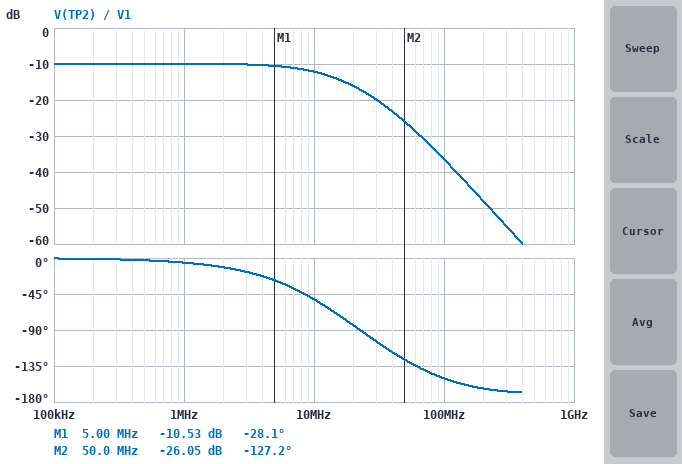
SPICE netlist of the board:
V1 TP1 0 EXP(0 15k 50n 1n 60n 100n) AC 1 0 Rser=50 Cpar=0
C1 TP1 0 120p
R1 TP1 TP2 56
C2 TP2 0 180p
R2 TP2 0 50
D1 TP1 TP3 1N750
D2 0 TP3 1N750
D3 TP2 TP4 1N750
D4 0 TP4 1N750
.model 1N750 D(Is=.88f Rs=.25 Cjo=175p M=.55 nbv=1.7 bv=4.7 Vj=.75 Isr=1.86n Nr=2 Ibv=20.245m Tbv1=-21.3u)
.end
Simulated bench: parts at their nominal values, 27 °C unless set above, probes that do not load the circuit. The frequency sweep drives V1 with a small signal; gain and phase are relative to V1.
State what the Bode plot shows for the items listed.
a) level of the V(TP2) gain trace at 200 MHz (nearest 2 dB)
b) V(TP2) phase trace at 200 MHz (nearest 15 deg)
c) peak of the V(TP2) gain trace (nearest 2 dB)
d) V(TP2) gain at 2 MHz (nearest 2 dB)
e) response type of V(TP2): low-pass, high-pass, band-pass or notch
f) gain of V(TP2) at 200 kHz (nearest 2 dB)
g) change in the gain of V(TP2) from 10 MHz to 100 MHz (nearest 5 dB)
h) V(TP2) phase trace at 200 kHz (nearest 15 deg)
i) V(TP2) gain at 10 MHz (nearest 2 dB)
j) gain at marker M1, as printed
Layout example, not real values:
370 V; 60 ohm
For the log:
-48 dB; -165 deg; -10 dB; -10 dB; low-pass; -10 dB; -25 dB; 0 deg; -12 dB; -10.53 dB
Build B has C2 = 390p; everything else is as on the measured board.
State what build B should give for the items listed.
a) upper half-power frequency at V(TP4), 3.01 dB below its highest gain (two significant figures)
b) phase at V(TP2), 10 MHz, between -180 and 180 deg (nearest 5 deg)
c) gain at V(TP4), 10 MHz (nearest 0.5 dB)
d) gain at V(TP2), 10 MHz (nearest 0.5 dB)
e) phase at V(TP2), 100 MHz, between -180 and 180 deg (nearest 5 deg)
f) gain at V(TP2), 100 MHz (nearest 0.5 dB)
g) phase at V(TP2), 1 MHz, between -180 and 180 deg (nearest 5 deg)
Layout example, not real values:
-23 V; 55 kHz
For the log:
8.1 MHz; -65 deg; -20.0 dB; -14.0 dB; -155 deg; -41.5 dB; -10 deg
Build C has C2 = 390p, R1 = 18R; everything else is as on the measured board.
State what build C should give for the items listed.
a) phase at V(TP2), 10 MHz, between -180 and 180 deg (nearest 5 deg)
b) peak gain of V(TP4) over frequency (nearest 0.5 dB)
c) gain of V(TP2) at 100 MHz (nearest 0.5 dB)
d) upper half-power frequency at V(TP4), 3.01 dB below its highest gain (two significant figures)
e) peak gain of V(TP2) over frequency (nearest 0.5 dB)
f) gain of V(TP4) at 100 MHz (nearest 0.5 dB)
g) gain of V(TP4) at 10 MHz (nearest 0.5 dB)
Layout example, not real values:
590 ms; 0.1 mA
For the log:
-55 deg; -13.5 dB; -33.0 dB; 8.9 MHz; -7.5 dB; -39.0 dB; -17.0 dB
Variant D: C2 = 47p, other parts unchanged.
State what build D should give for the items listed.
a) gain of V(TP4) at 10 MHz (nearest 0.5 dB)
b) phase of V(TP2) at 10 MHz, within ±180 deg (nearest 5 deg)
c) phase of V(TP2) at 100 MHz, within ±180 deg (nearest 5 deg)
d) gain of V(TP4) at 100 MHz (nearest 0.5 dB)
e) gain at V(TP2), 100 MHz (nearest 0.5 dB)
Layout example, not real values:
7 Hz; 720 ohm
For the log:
-17.0 dB; -40 deg; -140 deg; -37.0 dB; -31.0 dB
